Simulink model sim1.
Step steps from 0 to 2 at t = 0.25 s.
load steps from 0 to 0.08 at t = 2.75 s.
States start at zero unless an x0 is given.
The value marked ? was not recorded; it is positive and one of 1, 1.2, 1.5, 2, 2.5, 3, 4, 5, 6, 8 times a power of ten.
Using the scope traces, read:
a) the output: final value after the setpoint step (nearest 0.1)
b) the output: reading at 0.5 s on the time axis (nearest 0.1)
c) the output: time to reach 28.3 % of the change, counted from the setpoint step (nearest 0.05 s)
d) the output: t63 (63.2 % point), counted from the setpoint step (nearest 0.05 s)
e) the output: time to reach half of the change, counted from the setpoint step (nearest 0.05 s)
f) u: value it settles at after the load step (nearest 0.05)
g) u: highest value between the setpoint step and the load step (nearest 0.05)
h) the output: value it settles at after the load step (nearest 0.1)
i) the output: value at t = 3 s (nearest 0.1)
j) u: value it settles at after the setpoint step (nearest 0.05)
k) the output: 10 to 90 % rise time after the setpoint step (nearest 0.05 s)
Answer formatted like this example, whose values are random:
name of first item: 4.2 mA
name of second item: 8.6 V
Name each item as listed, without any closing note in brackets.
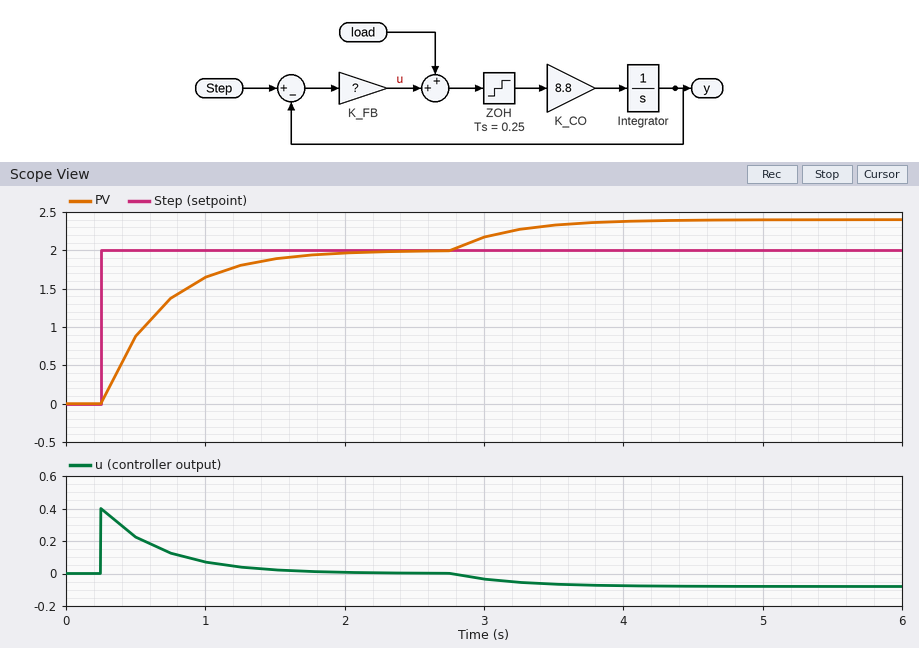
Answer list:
the output: final value after the setpoint step: 2.0
the output: reading at 0.5 s on the time axis: 0.9
the output: time to reach 28.3 % of the change, counted from the setpoint step: 0.15 s
the output: t63 (63.2 % point), counted from the setpoint step: 0.45 s
the output: time to reach half of the change, counted from the setpoint step: 0.30 s
u: value it settles at after the load step: -0.10
u: highest value between the setpoint step and the load step: 0.40
the output: value it settles at after the load step: 2.4
the output: value at t = 3 s: 2.2
u: value it settles at after the setpoint step: 0.00
the output: 10 to 90 % rise time after the setpoint step: 0.95 s
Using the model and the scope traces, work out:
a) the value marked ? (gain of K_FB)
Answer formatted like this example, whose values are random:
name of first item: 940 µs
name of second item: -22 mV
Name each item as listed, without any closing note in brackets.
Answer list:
the value marked ?: 0.2
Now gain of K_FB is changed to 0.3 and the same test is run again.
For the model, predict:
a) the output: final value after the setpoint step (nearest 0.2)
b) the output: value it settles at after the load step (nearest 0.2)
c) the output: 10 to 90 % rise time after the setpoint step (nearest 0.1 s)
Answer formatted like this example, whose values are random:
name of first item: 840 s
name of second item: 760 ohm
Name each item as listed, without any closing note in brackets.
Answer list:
the output: final value after the setpoint step: 2.0
the output: value it settles at after the load step: 2.2
the output: 10 to 90 % rise time after the setpoint step: 0.5 s
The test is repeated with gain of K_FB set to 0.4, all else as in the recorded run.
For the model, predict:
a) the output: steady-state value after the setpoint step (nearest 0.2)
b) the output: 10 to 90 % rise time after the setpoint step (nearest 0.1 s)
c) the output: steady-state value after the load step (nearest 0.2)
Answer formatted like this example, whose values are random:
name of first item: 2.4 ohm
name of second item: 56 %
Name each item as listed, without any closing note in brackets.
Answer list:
the output: steady-state value after the setpoint step: 2.0
the output: 10 to 90 % rise time after the setpoint step: 0.3 s
the output: steady-state value after the load step: 2.2
